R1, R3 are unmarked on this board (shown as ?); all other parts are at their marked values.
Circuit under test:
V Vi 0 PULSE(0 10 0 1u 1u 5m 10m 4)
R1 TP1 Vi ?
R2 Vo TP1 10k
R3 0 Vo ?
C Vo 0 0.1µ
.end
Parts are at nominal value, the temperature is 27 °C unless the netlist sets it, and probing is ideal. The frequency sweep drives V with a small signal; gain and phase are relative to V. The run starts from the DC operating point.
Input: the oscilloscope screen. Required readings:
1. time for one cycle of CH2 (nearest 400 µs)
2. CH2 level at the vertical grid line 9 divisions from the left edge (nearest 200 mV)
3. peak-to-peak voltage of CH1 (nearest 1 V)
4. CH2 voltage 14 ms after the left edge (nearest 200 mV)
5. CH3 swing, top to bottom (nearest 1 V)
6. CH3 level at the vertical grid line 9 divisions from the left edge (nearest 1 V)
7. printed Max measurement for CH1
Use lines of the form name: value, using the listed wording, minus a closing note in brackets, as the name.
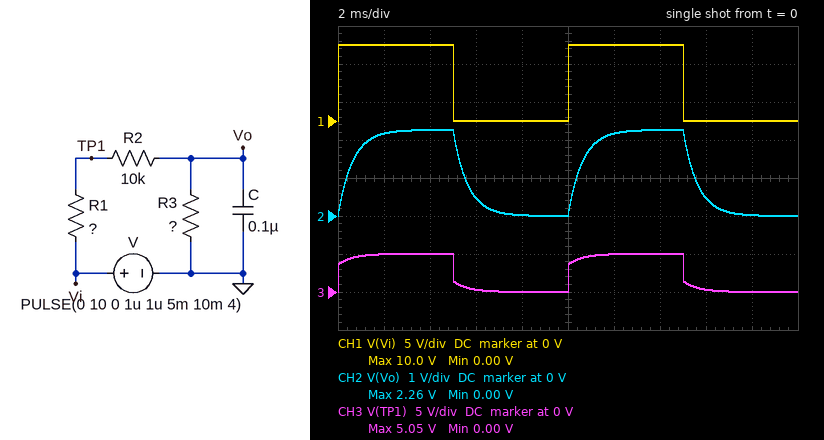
time for one cycle of CH2: 10.0 ms
CH2 level at the vertical grid line 9 divisions from the left edge: 0 V
peak-to-peak voltage of CH1: 10 V
CH2 voltage 14 ms after the left edge: 2.2 V
CH3 swing, top to bottom: 5 V
CH3 level at the vertical grid line 9 divisions from the left edge: 0 V
printed Max measurement for CH1: 10.0 V
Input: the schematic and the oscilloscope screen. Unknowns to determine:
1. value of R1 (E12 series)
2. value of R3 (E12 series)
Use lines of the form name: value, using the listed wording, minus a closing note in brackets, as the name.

value of R1: 18 kΩ
value of R3: 8.2 kΩ
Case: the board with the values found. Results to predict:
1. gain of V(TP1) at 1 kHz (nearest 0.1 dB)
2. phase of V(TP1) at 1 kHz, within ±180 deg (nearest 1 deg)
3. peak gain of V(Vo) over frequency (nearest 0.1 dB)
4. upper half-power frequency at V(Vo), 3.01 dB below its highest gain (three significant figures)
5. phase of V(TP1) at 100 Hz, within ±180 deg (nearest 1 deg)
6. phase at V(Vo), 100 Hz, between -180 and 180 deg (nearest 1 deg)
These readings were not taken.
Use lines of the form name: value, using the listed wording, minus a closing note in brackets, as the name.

gain of V(TP1) at 1 kHz: -8.7 dB
phase of V(TP1) at 1 kHz, within ±180 deg: -5 deg
peak gain of V(Vo) over frequency: -12.9 dB
upper half-power frequency at V(Vo), 3.01 dB below its highest gain: 251 Hz
phase of V(TP1) at 100 Hz, within ±180 deg: -6 deg
phase at V(Vo), 100 Hz, between -180 and 180 deg: -22 deg
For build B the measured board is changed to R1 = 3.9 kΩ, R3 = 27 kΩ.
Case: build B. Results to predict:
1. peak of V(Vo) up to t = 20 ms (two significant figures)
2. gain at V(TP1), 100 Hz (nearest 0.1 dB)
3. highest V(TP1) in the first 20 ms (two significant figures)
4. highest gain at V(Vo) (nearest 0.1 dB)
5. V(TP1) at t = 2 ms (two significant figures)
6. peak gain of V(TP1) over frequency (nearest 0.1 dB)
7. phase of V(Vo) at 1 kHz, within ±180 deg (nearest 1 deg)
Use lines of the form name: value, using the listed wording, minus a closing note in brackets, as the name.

peak of V(Vo) up to t = 20 ms: 6.6 V
gain at V(TP1), 100 Hz: -1.3 dB
highest V(TP1) in the first 20 ms: 9.0 V
highest gain at V(Vo): -3.6 dB
V(TP1) at t = 2 ms: 8.8 V
peak gain of V(TP1) over frequency: -0.9 dB
phase of V(Vo) at 1 kHz, within ±180 deg: -80 deg
